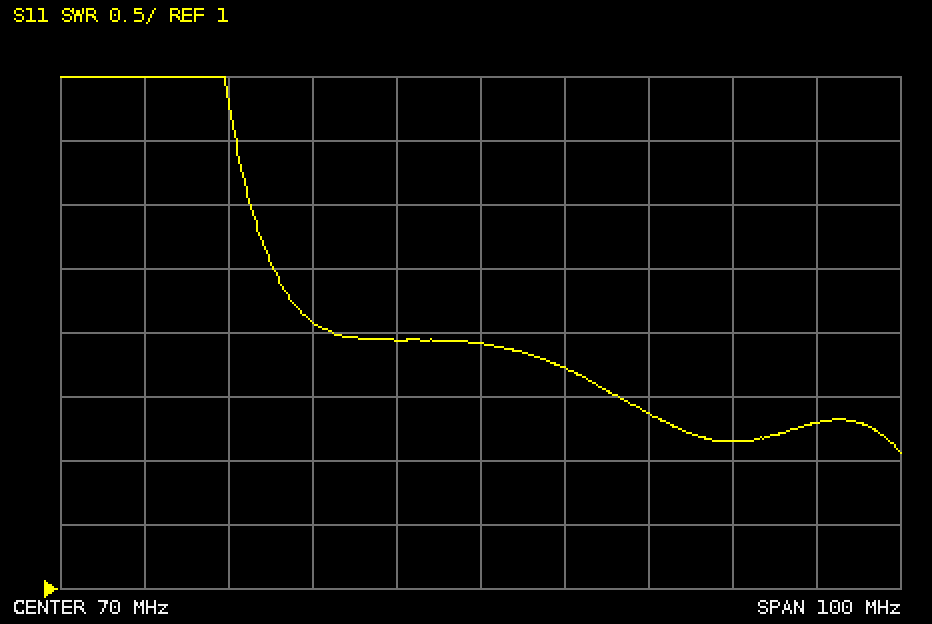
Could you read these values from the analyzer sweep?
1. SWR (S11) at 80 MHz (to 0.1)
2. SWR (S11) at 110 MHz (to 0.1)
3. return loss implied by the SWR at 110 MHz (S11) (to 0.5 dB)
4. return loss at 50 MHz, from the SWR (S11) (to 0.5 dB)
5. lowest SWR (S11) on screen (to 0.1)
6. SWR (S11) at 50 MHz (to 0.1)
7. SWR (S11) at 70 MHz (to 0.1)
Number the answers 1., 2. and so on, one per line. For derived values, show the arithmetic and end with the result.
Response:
1. 2.7
2. 2.3
3. −20 log10((2.3 − 1)/(2.3 + 1)) ≈ 8.09 dB, so 8.0 dB to the nearest 0.5 dB
4. −20 log10((3.1 − 1)/(3.1 + 1)) ≈ 5.81 dB, so 6.0 dB to the nearest 0.5 dB
5. 2.1
6. 3.1
7. 2.9
